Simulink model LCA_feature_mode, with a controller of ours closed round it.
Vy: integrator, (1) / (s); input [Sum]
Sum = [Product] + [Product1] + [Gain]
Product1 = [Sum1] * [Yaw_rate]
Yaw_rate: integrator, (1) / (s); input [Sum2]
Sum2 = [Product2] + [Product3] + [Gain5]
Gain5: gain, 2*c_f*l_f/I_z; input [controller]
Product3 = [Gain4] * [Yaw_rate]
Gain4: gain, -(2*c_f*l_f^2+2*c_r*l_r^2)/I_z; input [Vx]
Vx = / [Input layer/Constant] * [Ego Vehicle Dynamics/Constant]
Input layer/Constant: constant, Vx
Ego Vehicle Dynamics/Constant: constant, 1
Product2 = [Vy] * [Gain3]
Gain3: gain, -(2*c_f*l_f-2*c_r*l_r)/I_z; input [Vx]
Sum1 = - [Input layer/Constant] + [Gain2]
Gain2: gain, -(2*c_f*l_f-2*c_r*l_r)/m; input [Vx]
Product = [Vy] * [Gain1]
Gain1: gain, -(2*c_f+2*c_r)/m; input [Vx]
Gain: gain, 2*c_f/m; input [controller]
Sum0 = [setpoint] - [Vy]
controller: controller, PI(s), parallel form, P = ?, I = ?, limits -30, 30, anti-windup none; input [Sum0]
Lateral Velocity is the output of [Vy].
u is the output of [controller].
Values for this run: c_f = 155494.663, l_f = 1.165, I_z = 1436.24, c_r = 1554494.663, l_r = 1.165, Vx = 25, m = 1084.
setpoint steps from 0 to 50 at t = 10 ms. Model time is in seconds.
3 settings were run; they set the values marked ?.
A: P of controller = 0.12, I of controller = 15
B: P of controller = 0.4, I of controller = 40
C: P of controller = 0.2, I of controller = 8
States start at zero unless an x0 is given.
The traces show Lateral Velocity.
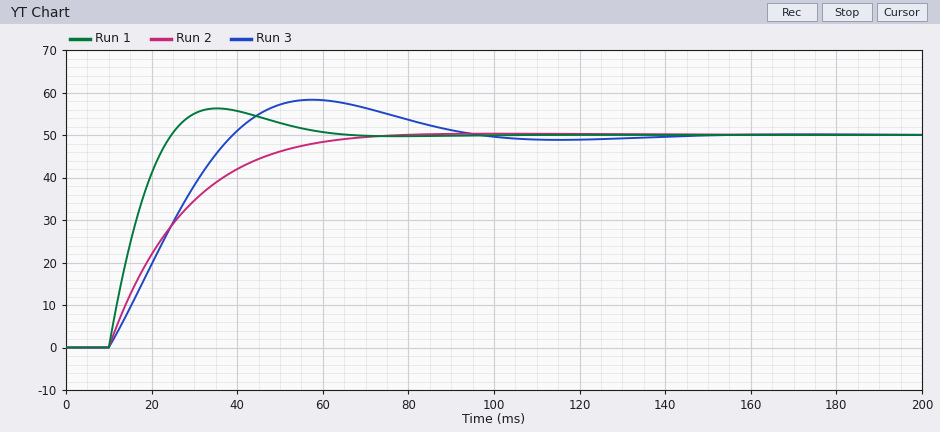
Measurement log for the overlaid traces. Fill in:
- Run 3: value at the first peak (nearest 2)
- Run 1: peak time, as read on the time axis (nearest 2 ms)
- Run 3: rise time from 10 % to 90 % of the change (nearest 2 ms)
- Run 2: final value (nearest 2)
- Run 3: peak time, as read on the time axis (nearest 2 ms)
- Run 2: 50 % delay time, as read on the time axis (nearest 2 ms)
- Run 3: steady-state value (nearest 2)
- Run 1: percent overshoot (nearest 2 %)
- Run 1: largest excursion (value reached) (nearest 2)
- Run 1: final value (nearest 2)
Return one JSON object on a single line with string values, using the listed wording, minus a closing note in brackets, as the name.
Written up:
{"Run 3: value at the first peak": "58", "Run 1: peak time, as read on the time axis": "36 ms", "Run 3: rise time from 10 % to 90 % of the change": "22 ms", "Run 2: final value": "50", "Run 3: peak time, as read on the time axis": "58 ms", "Run 2: 50 % delay time, as read on the time axis": "22 ms", "Run 3: steady-state value": "50", "Run 1: percent overshoot": "12 %", "Run 1: largest excursion (value reached)": "56", "Run 1: final value": "50"}
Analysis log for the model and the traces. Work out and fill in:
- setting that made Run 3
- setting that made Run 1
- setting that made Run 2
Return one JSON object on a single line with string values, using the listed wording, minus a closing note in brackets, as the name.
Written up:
{"setting that made Run 3": "A", "setting that made Run 1": "B", "setting that made Run 2": "C"}
